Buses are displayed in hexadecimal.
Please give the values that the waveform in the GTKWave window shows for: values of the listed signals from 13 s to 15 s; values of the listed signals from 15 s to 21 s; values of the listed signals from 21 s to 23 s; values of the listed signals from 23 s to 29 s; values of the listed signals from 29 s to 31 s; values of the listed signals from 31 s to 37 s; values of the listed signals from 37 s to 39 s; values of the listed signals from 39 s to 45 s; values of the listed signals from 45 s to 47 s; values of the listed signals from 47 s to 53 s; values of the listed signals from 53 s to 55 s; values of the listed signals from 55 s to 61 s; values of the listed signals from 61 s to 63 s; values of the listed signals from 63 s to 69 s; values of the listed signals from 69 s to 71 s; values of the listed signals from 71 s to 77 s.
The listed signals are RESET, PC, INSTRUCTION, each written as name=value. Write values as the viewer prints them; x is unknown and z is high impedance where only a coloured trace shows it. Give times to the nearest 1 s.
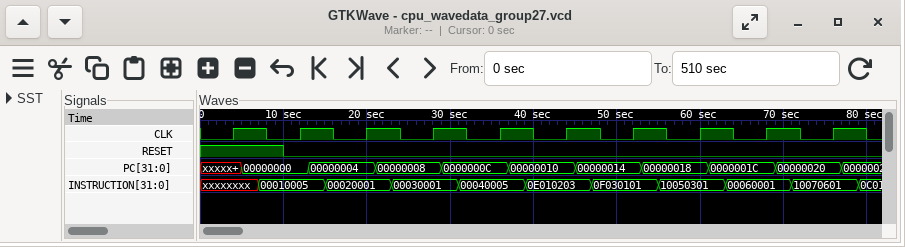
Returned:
RESET=0, PC=00000004, INSTRUCTION=00010005
RESET=0, PC=00000004, INSTRUCTION=00020001
RESET=0, PC=00000008, INSTRUCTION=00020001
RESET=0, PC=00000008, INSTRUCTION=00030001
RESET=0, PC=0000000C, INSTRUCTION=00030001
RESET=0, PC=0000000C, INSTRUCTION=00040005
RESET=0, PC=00000010, INSTRUCTION=00040005
RESET=0, PC=00000010, INSTRUCTION=0E010203
RESET=0, PC=00000014, INSTRUCTION=0E010203
RESET=0, PC=00000014, INSTRUCTION=0F030101
RESET=0, PC=00000018, INSTRUCTION=0F030101
RESET=0, PC=00000018, INSTRUCTION=10050301
RESET=0, PC=0000001C, INSTRUCTION=10050301
RESET=0, PC=0000001C, INSTRUCTION=00060001
RESET=0, PC=00000020, INSTRUCTION=00060001
RESET=0, PC=00000020, INSTRUCTION=10070601
